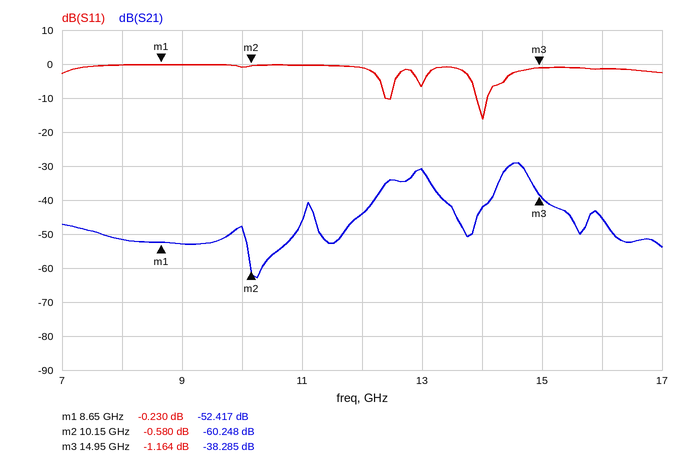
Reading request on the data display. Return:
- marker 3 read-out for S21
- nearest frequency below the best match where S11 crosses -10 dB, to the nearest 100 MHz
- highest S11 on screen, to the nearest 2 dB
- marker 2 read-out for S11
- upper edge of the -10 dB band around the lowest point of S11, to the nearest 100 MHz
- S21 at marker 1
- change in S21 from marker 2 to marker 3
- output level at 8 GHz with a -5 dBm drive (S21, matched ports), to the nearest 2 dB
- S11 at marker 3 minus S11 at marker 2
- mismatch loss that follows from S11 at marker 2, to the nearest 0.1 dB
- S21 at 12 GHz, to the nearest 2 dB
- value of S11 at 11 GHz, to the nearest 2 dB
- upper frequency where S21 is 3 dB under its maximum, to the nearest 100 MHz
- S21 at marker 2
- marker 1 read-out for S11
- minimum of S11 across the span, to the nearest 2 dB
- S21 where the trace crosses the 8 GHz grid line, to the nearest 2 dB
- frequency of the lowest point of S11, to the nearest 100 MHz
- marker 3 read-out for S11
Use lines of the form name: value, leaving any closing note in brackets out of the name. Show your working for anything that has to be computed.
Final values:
marker 3 read-out for S21: -38.285 dB
nearest frequency below the best match where S11 crosses -10 dB, to the nearest 100 MHz: 13.9 GHz
highest S11 on screen, to the nearest 2 dB: 0 dB
marker 2 read-out for S11: -0.580 dB
upper edge of the -10 dB band around the lowest point of S11, to the nearest 100 MHz: 14.1 GHz
S21 at marker 1: -52.417 dB
change in S21 from marker 2 to marker 3: -38.285 − (-60.248) = 21.963 dB
output level at 8 GHz with a -5 dBm drive (S21, matched ports), to the nearest 2 dB: -5 dBm + (-52 dB) = -56 dBm
S11 at marker 3 minus S11 at marker 2: -1.164 − (-0.58) = -0.584 dB
mismatch loss that follows from S11 at marker 2, to the nearest 0.1 dB: −10 log10(1 − 10^(-0.58/10)) ≈ 9.0 dB
S21 at 12 GHz, to the nearest 2 dB: -44 dB
value of S11 at 11 GHz, to the nearest 2 dB: 0 dB
upper frequency where S21 is 3 dB under its maximum, to the nearest 100 MHz: 14.7 GHz
S21 at marker 2: -60.248 dB
marker 1 read-out for S11: -0.230 dB
minimum of S11 across the span, to the nearest 2 dB: -16 dB
S21 where the trace crosses the 8 GHz grid line, to the nearest 2 dB: -52 dB
frequency of the lowest point of S11, to the nearest 100 MHz: 14.0 GHz
marker 3 read-out for S11: -1.164 dB
